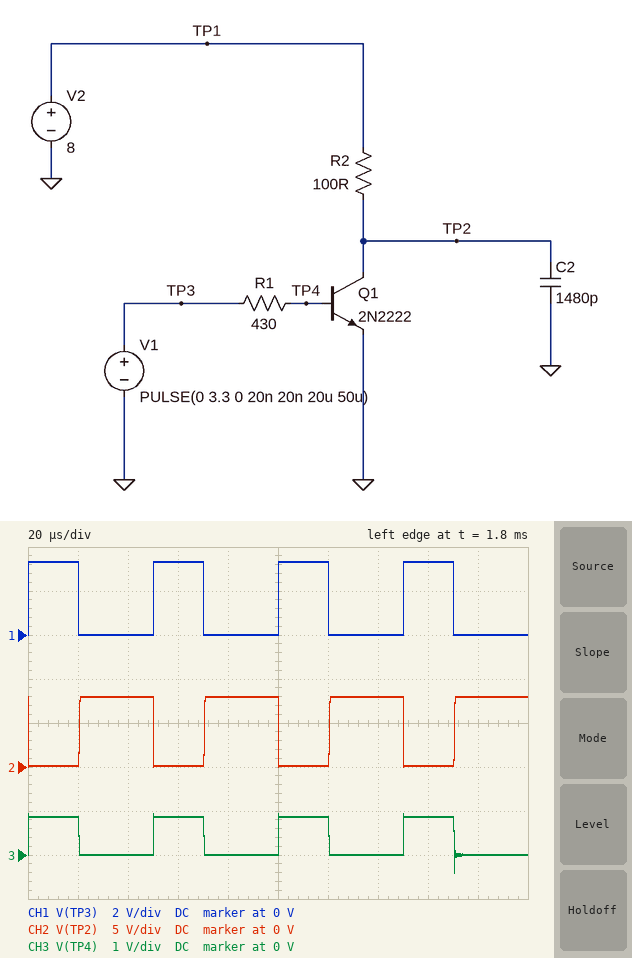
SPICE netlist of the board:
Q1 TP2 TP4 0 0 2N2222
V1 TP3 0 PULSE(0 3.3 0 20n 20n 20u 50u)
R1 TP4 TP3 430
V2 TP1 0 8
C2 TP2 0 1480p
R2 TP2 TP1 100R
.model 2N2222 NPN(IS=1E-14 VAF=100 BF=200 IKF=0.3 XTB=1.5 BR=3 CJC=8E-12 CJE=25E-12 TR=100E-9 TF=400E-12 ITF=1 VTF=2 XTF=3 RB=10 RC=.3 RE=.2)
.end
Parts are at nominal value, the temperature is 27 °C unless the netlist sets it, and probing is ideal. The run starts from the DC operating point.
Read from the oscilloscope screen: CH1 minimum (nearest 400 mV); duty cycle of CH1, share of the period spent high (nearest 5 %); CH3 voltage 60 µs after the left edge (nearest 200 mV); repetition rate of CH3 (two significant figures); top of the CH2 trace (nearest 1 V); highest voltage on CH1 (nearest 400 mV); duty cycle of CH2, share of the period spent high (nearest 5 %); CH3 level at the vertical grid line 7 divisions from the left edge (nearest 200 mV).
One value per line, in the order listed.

0 V
40 %
800 mV
20 kHz
8 V
3.2 V
60 %
0 V
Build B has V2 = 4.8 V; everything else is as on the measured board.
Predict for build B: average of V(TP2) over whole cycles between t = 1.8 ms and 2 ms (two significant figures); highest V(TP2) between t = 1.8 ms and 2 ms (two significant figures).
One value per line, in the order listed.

2.9 V
4.8 V
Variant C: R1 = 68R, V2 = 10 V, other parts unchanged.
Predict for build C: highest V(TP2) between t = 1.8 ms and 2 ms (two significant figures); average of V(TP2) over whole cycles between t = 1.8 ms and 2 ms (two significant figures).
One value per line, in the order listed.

10 V
5.9 V
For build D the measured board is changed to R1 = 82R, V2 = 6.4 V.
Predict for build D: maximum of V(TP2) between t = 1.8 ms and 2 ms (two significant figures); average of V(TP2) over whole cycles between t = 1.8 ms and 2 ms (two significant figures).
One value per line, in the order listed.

6.4 V
3.8 V
